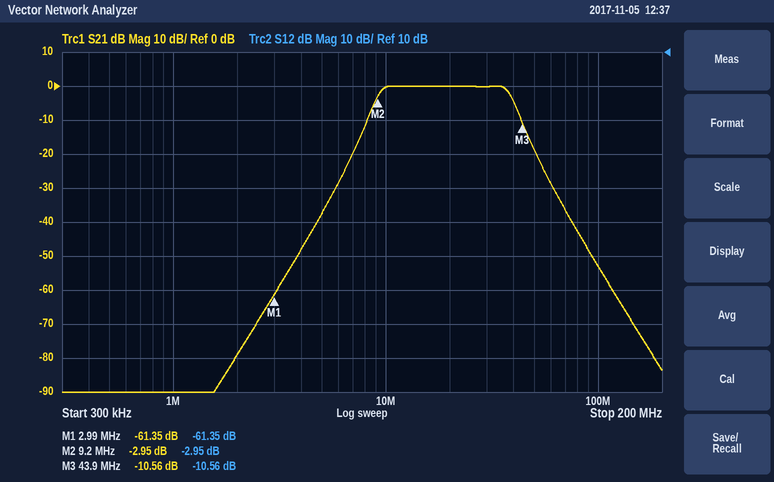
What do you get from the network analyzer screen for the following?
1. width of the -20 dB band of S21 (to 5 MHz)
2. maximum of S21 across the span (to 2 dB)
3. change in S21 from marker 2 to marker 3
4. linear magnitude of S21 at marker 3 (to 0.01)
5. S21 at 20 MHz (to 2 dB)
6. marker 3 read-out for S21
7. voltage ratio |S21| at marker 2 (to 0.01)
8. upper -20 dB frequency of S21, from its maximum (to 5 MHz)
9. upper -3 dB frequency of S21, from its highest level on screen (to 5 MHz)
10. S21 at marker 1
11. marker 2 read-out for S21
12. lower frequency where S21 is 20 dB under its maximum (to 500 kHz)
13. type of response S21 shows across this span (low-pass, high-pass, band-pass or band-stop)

45 MHz
0 dB
-7.61 dB
0.30
0 dB
-10.56 dB
0.71
50 MHz
40 MHz
-61.35 dB
-2.95 dB
7.0 MHz
band-pass
